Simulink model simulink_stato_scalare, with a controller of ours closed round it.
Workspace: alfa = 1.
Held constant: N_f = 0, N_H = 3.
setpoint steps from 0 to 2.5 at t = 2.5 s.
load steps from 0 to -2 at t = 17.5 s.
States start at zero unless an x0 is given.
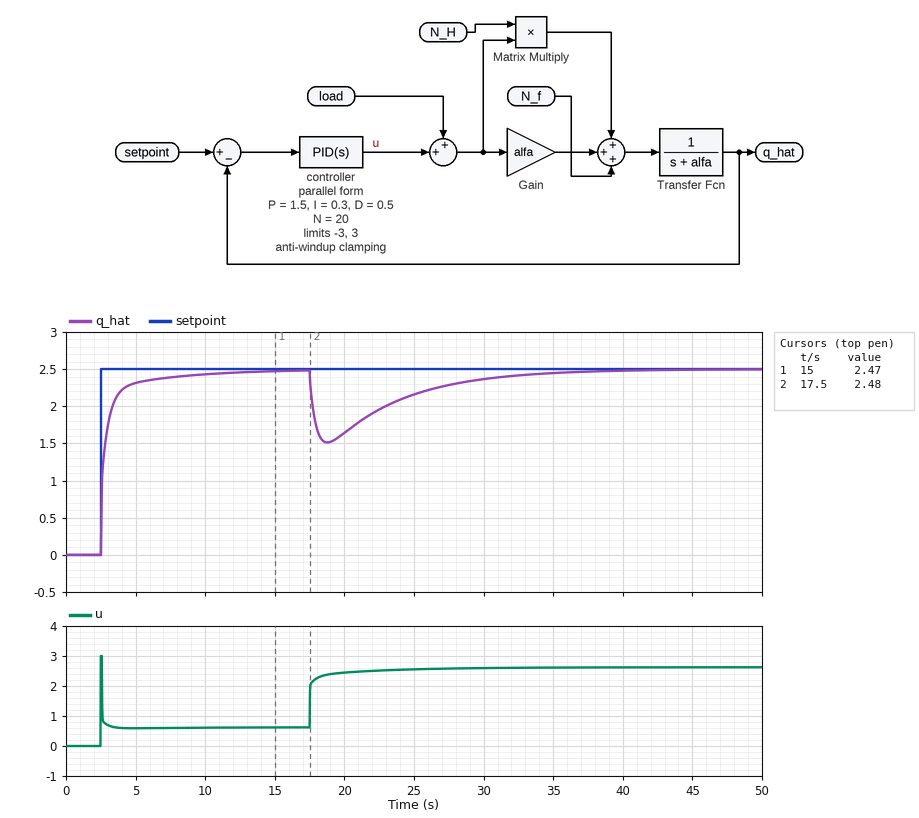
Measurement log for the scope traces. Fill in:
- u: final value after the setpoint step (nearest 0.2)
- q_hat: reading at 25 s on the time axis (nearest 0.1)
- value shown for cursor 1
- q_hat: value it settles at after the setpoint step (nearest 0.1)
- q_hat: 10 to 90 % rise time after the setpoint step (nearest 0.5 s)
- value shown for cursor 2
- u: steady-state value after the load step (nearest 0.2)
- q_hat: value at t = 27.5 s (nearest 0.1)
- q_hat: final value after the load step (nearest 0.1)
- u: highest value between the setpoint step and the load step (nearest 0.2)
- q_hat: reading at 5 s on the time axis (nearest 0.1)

0.6
2.2
2.47
2.5
1.5 s
2.48
2.6
2.3
2.5
3.0
2.3
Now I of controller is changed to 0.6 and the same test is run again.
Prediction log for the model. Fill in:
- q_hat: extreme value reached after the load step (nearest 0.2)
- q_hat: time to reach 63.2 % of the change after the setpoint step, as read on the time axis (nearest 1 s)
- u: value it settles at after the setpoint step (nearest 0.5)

1.6
3 s
0.5
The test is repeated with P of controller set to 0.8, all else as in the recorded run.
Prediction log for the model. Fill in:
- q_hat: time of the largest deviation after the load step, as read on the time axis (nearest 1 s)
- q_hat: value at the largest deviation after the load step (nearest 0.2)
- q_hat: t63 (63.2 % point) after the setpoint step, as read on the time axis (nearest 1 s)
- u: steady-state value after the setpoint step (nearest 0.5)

19 s
1.0
3 s
0.5
